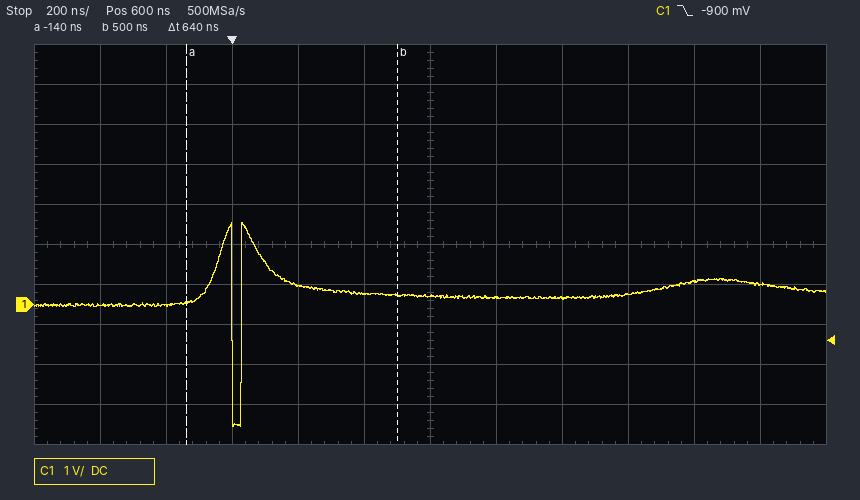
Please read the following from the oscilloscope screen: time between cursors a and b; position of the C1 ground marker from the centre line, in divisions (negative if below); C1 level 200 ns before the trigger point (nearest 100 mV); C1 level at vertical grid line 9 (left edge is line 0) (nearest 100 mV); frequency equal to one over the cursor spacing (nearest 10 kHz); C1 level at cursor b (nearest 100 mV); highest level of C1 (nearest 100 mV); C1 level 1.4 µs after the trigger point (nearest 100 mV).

640 ns
-1.5 div
0.0 V
300 mV
1.56 MHz
200 mV
2.0 V
600 mV
